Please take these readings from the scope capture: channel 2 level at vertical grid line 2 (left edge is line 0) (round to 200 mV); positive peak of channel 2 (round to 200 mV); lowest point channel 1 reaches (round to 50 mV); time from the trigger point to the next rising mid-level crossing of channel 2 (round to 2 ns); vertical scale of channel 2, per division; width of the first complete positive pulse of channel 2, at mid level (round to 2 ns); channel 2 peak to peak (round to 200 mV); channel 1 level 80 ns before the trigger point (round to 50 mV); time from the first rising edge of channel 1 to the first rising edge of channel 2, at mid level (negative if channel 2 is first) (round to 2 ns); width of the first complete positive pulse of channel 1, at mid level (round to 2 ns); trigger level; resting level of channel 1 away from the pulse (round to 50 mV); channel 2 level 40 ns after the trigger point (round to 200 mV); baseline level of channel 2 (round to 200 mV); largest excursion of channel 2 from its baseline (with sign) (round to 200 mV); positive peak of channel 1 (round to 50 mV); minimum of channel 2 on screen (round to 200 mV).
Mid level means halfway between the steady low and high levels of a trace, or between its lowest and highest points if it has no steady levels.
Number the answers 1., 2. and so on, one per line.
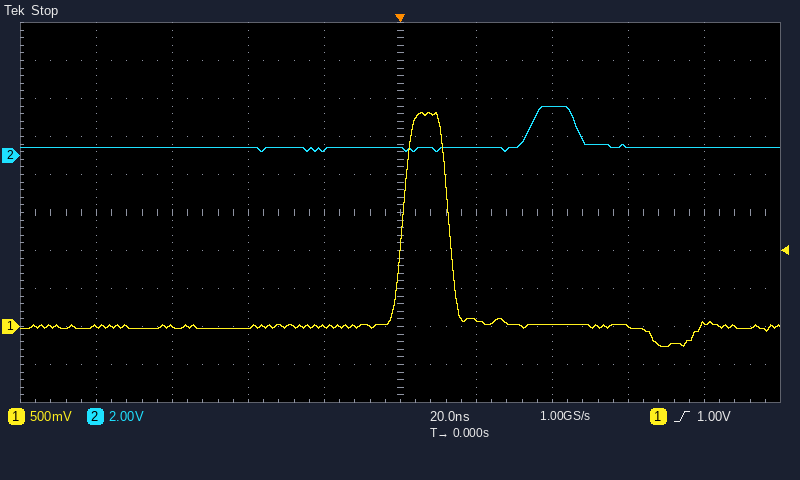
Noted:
1. 400 mV
2. 2.6 V
3. -250 mV
4. 34 ns
5. 2 V
6. 12 ns
7. 2.4 V
8. 0 mV
9. +34 ns
10. 12 ns
11. 1.00 V
12. 0 mV
13. 2.6 V
14. 400 mV
15. +2.2 V
16. 2.80 V
17. 200 mV
